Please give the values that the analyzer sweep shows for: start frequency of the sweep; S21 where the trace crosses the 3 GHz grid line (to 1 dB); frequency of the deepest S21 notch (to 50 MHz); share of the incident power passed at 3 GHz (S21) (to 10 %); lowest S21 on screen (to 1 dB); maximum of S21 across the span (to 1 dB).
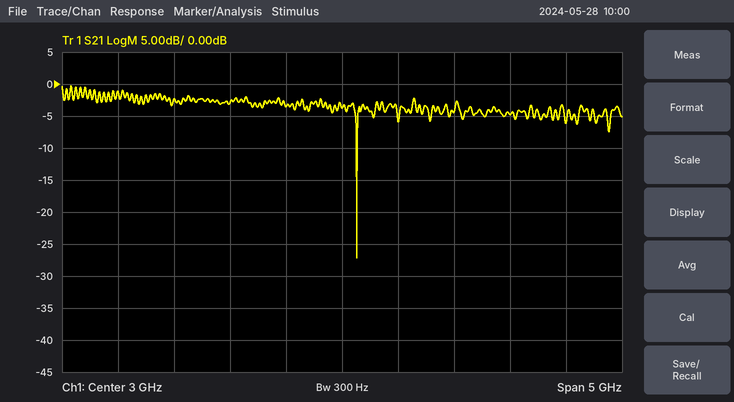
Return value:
500 MHz
-4 dB
3.15 GHz
40 %
-27 dB
0 dB
